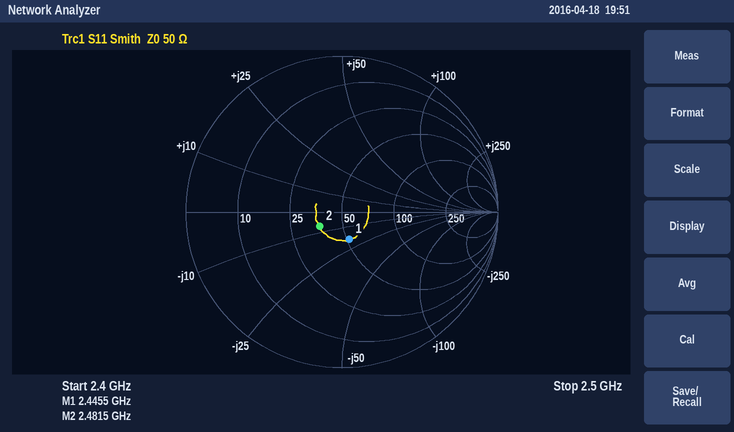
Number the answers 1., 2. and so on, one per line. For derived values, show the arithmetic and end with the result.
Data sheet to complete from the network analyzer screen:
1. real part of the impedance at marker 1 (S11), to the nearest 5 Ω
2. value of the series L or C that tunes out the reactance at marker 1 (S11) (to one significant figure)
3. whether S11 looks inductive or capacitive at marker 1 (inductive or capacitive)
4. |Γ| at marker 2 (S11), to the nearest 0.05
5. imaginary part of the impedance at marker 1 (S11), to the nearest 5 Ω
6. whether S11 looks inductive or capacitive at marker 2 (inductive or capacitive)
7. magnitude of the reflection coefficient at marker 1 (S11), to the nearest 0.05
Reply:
1. 50 Ω
2. L = 20 Ω/(2π × 2.4455 GHz) ≈ 1 nH
3. capacitive
4. 0.15
5. -20 Ω
6. capacitive
7. 0.20
